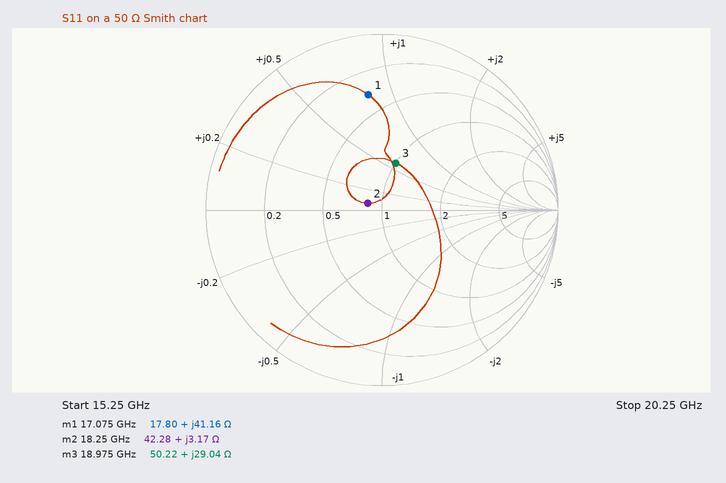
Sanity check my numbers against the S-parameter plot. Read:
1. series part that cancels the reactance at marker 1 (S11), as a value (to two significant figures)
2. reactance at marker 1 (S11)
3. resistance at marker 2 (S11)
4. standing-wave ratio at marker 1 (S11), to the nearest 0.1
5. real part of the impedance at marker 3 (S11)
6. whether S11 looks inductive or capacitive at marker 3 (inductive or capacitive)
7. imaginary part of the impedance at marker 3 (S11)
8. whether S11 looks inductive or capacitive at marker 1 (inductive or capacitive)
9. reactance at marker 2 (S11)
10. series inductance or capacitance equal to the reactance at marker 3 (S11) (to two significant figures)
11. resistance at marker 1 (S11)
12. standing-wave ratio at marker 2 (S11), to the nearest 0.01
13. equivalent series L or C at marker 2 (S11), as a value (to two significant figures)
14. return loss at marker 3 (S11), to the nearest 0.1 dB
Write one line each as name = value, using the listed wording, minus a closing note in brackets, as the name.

series part that cancels the reactance at marker 1 (S11), as a value = 230 fF
reactance at marker 1 = +41.16 Ω
resistance at marker 2 = 42.28 Ω
standing-wave ratio at marker 1 (S11), to the nearest 0.1 = 4.9
real part of the impedance at marker 3 = 50.22 Ω
whether S11 looks inductive or capacitive at marker 3 = inductive
imaginary part of the impedance at marker 3 = +29.04 Ω
whether S11 looks inductive or capacitive at marker 1 = inductive
reactance at marker 2 = +3.17 Ω
series inductance or capacitance equal to the reactance at marker 3 (S11) = 240 pH
resistance at marker 1 = 17.80 Ω
standing-wave ratio at marker 2 (S11), to the nearest 0.01 = 1.20
equivalent series L or C at marker 2 (S11), as a value = 28 pH
return loss at marker 3 (S11), to the nearest 0.1 dB = 11.1 dB
